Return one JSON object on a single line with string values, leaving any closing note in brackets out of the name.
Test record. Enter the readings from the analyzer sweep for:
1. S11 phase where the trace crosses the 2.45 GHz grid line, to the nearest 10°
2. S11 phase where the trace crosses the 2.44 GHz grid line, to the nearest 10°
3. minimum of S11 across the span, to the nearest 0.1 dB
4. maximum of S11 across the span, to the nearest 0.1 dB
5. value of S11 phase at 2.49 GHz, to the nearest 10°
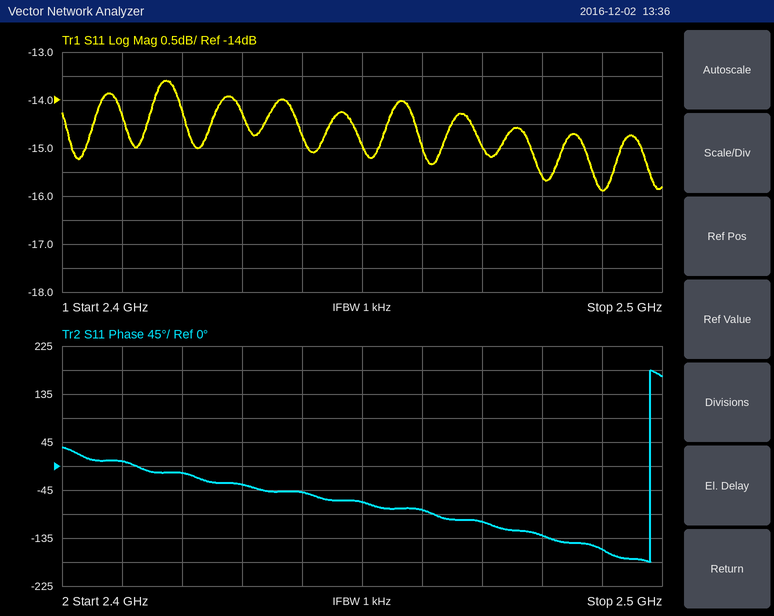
{"S11 phase where the trace crosses the 2.45 GHz grid line, to the nearest 10°": "-70°", "S11 phase where the trace crosses the 2.44 GHz grid line, to the nearest 10°": "-50°", "minimum of S11 across the span, to the nearest 0.1 dB": "-15.9 dB", "maximum of S11 across the span, to the nearest 0.1 dB": "-13.6 dB", "value of S11 phase at 2.49 GHz, to the nearest 10°": "-160°"}
